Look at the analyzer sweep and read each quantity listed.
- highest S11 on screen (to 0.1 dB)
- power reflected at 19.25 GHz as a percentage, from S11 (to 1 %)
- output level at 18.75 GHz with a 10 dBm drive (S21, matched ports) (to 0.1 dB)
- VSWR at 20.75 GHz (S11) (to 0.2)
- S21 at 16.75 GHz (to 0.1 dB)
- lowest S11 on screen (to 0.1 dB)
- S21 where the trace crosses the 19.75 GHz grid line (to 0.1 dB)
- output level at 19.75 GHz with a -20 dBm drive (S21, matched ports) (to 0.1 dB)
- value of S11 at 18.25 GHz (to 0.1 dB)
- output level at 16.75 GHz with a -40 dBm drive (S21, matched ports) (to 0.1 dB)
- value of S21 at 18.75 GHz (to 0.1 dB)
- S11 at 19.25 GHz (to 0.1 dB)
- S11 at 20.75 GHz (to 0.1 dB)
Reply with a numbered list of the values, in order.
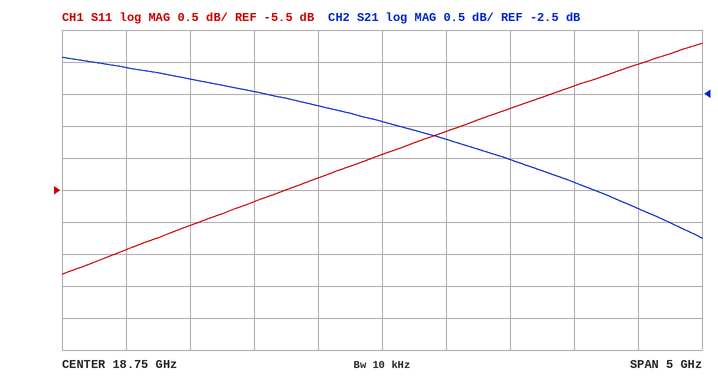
1. -3.2 dB
2. 35 %
3. 7.1 dBm
4. 5.0
5. -2.1 dB
6. -6.8 dB
7. -3.5 dB
8. -23.5 dBm
9. -5.3 dB
10. -42.1 dBm
11. -2.9 dB
12. -4.6 dB
13. -3.5 dB
